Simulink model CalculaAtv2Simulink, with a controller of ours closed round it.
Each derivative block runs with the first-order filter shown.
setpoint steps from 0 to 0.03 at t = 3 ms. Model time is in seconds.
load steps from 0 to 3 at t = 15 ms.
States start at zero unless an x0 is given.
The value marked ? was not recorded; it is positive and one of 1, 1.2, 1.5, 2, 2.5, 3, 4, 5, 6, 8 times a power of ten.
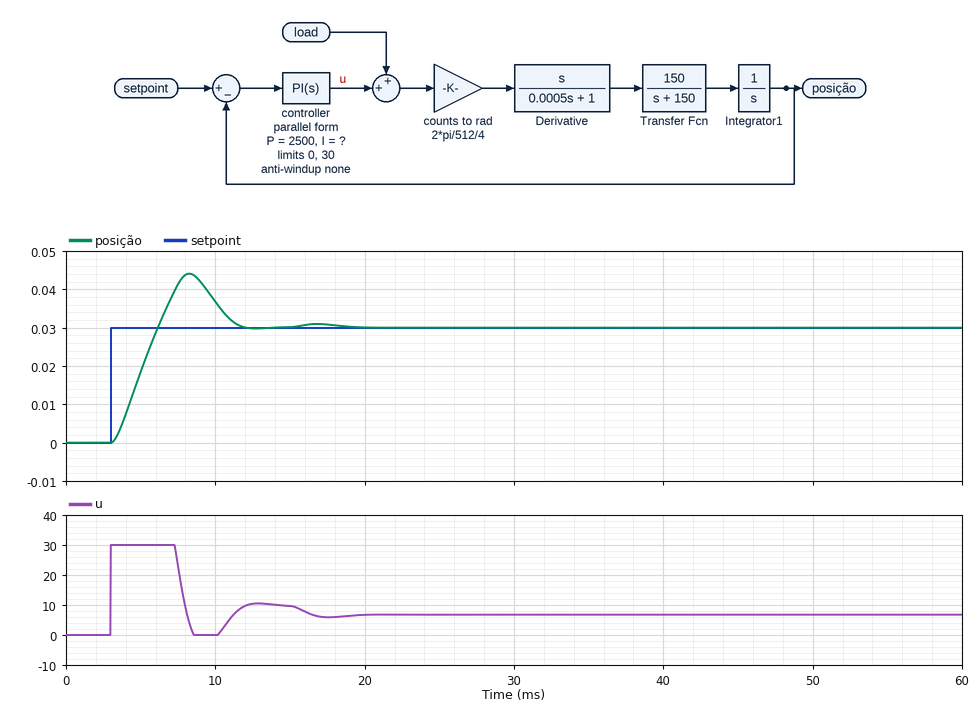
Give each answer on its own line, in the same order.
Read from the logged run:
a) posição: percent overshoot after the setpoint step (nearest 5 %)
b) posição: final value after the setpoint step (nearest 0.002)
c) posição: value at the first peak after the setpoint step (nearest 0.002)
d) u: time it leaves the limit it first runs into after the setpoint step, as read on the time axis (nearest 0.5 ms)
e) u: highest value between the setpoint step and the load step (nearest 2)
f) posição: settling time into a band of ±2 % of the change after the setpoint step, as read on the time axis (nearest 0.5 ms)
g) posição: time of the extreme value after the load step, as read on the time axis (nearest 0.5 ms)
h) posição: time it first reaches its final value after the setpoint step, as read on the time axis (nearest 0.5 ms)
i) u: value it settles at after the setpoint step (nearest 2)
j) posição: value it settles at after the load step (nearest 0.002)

45 %
0.030
0.044
7.5 ms
30
11.5 ms
17.0 ms
6.0 ms
10
0.030
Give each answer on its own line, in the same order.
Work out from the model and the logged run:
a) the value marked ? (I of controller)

1.2e+06
